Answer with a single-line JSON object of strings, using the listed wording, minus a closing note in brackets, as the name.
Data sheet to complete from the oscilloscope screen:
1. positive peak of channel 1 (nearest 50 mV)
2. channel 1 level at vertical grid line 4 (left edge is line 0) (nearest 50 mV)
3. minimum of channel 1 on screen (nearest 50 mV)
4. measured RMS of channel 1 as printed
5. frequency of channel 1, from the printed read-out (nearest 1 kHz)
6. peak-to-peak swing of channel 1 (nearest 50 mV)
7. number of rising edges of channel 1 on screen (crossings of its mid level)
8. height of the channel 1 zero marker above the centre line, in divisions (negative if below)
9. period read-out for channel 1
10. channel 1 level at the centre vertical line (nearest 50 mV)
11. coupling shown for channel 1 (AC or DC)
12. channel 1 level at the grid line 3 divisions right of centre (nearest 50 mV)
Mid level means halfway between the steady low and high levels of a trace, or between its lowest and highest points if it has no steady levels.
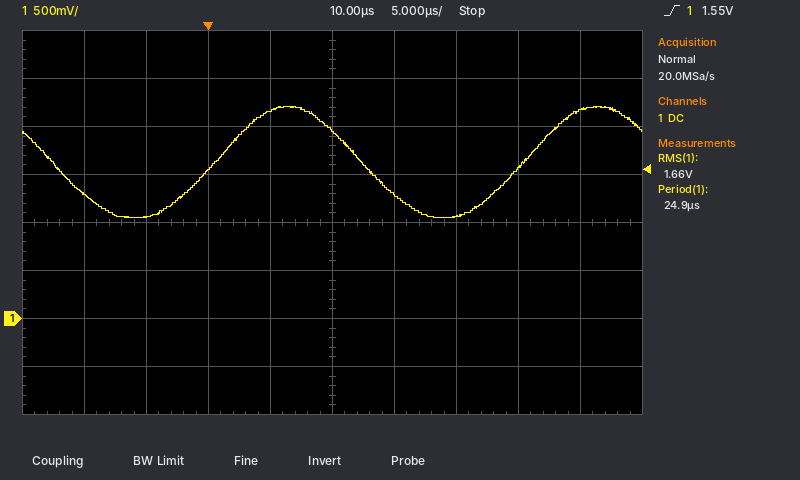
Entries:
{"positive peak of channel 1": "2.20 V", "channel 1 level at vertical grid line 4 (left edge is line 0)": "2.15 V", "minimum of channel 1 on screen": "1.05 V", "measured RMS of channel 1 as printed": "1.66 V", "frequency of channel 1, from the printed read-out": "40 kHz", "peak-to-peak swing of channel 1": "1.15 V", "number of rising edges of channel 1 on screen": "2", "height of the channel 1 zero marker above the centre line, in divisions": "-2.0 div", "period read-out for channel 1": "24.9 µs", "channel 1 level at the centre vertical line": "1.95 V", "coupling shown for channel 1": "DC", "channel 1 level at the grid line 3 divisions right of centre": "1.55 V"}
